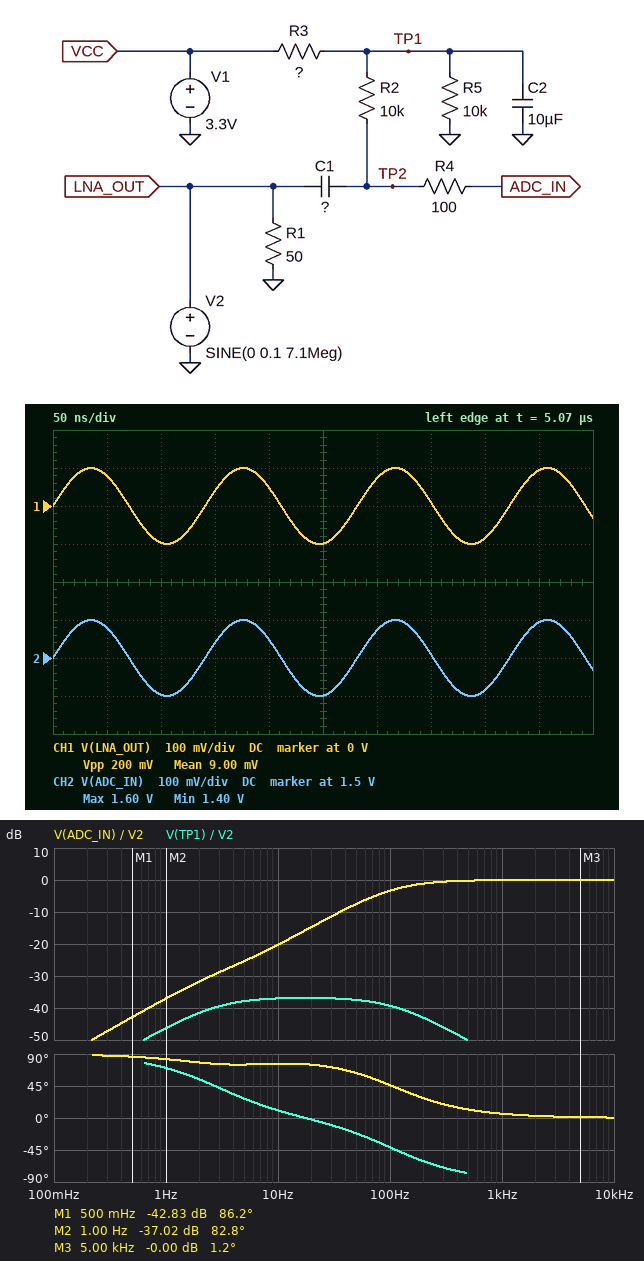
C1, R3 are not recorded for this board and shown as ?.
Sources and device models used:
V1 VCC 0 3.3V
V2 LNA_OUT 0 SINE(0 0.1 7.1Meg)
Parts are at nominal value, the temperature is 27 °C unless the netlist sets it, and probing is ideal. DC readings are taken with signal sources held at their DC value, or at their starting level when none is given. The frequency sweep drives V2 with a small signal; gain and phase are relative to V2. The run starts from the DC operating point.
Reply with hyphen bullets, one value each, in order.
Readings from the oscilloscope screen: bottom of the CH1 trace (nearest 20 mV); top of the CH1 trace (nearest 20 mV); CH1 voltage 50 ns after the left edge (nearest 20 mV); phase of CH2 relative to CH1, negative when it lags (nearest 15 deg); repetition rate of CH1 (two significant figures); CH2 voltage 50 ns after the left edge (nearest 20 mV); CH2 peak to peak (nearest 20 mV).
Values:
- -100 mV
- 100 mV
- 80 mV
- 0 deg
- 7.1 MHz
- 1.58 V
- 200 mV
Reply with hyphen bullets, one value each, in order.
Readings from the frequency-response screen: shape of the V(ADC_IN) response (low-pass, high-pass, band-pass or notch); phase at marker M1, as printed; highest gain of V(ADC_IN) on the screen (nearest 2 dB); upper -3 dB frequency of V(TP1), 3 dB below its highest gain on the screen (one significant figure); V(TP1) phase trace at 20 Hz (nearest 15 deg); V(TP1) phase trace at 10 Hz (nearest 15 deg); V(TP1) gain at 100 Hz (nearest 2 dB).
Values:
- high-pass
- 86.2 deg
- 0 dB
- 100 Hz
- 0 deg
- 15 deg
- -40 dB
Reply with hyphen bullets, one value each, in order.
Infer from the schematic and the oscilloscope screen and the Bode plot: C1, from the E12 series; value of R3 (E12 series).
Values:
- 150 nF
- 12 kΩ
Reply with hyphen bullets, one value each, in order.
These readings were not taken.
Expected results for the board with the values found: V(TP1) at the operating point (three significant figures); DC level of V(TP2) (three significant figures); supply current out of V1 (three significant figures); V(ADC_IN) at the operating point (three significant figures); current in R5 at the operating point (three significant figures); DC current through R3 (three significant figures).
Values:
- 1.50 V
- 1.50 V
- 150 µA
- 1.50 V
- 150 µA
- 150 µA
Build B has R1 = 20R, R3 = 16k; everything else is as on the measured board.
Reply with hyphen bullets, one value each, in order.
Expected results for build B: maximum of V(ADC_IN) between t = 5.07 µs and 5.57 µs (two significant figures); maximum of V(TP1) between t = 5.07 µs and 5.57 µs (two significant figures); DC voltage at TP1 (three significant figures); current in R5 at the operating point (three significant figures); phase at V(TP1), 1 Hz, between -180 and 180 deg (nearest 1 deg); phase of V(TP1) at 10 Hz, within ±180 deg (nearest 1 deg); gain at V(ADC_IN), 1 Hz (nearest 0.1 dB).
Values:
- 1.4 V
- 1.3 V
- 1.27 V
- 127 µA
- 68 deg
- 9 deg
- -36.7 dB
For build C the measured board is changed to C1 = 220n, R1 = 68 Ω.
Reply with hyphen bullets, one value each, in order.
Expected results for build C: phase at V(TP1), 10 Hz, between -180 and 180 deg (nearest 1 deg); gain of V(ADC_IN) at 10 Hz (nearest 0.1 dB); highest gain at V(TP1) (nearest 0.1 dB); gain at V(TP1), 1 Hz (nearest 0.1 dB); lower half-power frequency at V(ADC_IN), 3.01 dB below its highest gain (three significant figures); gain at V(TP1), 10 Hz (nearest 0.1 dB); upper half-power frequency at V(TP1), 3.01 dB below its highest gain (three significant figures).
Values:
- 8 deg
- -17.0 dB
- -33.7 dB
- -43.0 dB
- 73.8 Hz
- -33.8 dB
- 79.5 Hz
